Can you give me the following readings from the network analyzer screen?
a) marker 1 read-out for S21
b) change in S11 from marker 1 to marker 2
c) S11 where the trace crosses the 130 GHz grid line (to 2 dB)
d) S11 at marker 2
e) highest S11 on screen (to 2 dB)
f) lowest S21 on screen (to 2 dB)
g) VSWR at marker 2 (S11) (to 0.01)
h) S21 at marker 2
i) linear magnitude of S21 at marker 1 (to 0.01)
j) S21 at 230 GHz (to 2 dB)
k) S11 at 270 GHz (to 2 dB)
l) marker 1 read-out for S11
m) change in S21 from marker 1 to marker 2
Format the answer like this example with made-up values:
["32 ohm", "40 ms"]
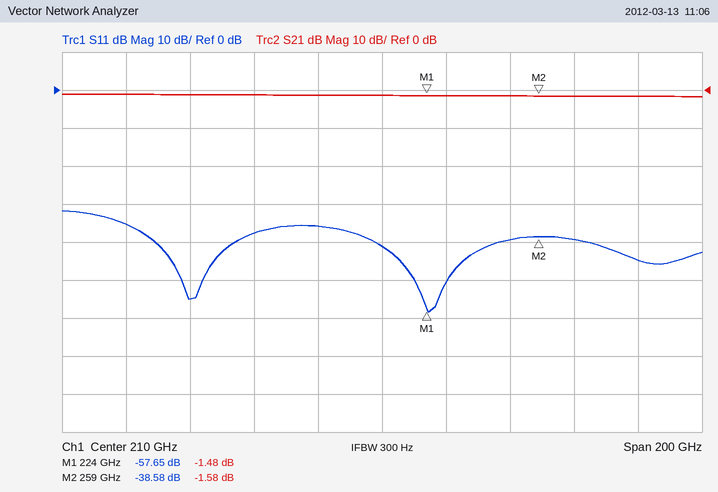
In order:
["-1.48 dB", "19.07 dB", "-36 dB", "-38.58 dB", "-32 dB", "-2 dB", "1.02", "-1.58 dB", "0.84", "-2 dB", "-40 dB", "-57.65 dB", "-0.10 dB"]
